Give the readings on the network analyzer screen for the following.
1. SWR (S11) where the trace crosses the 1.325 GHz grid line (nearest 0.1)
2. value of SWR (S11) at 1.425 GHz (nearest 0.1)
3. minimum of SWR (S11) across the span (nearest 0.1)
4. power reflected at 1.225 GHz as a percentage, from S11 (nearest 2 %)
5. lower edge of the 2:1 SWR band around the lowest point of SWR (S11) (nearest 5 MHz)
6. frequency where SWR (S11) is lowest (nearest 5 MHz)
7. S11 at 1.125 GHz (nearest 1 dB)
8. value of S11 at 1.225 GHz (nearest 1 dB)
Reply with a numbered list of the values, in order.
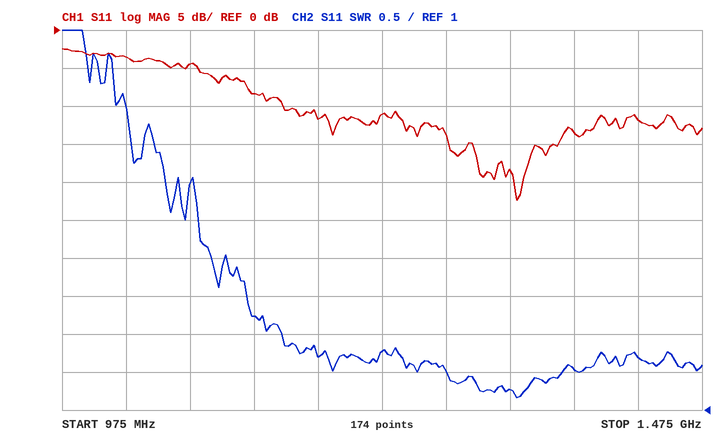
1. 1.3
2. 1.7
3. 1.2
4. 8 %
5. 1.145 GHz
6. 1.330 GHz
7. -8 dB
8. -11 dB
